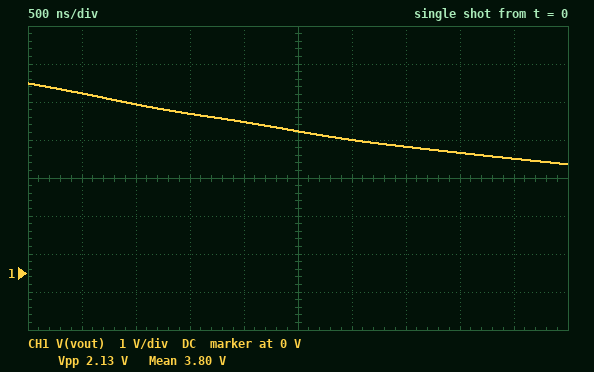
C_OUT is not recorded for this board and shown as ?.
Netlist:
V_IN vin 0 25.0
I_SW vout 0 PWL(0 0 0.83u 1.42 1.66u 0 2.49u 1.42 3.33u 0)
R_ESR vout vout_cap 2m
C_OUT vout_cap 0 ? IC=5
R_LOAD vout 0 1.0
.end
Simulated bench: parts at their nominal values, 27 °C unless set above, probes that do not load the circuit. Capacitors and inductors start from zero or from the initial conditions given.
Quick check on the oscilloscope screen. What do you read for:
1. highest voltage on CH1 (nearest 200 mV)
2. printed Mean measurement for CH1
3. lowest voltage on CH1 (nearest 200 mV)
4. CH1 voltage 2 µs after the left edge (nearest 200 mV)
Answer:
5.0 V
3.80 V
2.8 V
4.0 V
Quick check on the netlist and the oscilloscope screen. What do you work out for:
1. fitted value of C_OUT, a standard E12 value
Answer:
10 µF
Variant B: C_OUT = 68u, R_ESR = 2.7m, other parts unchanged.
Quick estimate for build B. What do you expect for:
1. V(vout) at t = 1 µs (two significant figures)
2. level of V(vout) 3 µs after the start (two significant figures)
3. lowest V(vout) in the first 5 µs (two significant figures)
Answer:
4.9 V
4.7 V
4.6 V
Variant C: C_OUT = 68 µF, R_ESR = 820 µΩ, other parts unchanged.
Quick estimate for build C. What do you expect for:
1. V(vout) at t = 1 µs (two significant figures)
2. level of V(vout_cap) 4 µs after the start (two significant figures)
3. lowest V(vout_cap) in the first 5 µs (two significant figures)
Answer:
4.9 V
4.7 V
4.6 V
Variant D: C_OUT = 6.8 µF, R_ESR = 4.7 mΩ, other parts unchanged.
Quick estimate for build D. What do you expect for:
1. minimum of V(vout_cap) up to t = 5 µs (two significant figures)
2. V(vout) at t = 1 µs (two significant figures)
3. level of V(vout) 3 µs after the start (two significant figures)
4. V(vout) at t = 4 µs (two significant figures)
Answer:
2.2 V
4.2 V
2.9 V
2.5 V
